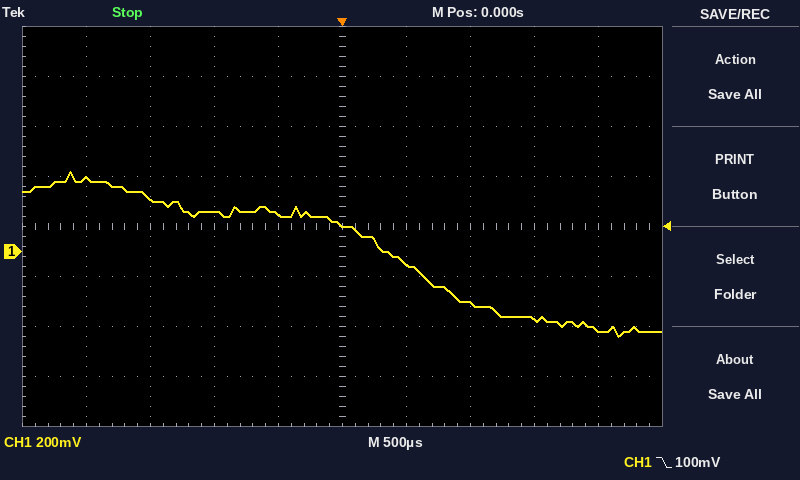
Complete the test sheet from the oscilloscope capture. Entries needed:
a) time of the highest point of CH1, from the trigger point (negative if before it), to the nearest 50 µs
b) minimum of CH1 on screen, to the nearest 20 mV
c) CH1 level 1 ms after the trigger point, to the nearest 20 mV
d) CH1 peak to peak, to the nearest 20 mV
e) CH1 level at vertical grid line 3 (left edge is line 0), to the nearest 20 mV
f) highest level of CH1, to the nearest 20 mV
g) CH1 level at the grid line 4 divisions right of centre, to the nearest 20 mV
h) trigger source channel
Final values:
-2.10 ms
-340 mV
-200 mV
660 mV
160 mV
320 mV
-320 mV
CH1
